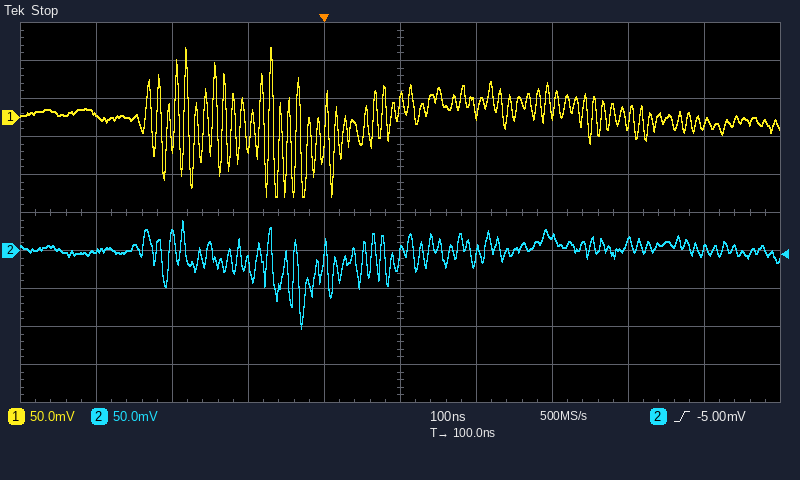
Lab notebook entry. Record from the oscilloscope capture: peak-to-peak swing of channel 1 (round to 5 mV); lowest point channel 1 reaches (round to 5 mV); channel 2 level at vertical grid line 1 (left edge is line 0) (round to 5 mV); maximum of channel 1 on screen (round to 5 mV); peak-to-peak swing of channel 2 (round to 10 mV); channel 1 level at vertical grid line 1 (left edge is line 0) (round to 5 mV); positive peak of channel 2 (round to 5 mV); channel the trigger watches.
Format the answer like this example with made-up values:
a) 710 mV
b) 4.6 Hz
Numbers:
a) 195 mV
b) -105 mV
c) 0 mV
d) 90 mV
e) 140 mV
f) 5 mV
g) 40 mV
h) channel 2
